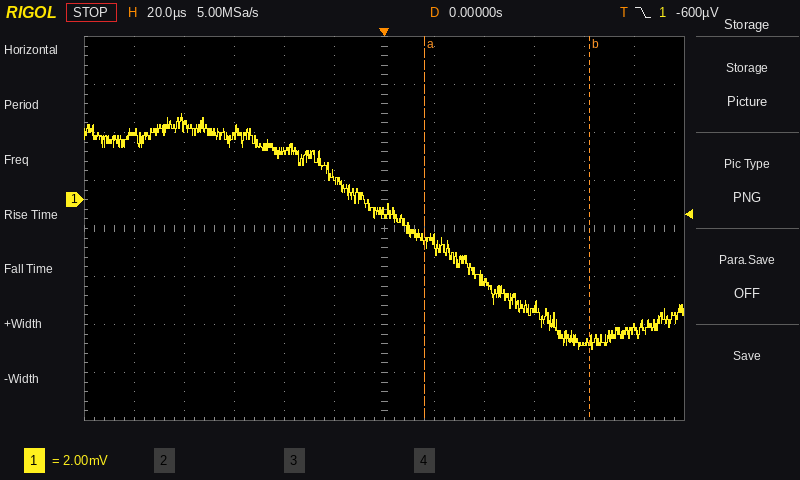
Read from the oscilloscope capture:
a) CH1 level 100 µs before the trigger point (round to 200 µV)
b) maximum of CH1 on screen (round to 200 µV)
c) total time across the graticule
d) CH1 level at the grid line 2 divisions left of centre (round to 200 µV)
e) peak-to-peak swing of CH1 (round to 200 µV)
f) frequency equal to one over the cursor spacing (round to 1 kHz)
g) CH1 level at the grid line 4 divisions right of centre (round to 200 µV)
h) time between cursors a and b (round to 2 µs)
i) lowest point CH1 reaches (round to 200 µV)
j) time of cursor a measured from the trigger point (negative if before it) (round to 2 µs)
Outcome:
2.8 mV
3.6 mV
240 µs
2.0 mV
9.8 mV
15 kHz
-6.0 mV
66 µs
-6.2 mV
+16 µs
